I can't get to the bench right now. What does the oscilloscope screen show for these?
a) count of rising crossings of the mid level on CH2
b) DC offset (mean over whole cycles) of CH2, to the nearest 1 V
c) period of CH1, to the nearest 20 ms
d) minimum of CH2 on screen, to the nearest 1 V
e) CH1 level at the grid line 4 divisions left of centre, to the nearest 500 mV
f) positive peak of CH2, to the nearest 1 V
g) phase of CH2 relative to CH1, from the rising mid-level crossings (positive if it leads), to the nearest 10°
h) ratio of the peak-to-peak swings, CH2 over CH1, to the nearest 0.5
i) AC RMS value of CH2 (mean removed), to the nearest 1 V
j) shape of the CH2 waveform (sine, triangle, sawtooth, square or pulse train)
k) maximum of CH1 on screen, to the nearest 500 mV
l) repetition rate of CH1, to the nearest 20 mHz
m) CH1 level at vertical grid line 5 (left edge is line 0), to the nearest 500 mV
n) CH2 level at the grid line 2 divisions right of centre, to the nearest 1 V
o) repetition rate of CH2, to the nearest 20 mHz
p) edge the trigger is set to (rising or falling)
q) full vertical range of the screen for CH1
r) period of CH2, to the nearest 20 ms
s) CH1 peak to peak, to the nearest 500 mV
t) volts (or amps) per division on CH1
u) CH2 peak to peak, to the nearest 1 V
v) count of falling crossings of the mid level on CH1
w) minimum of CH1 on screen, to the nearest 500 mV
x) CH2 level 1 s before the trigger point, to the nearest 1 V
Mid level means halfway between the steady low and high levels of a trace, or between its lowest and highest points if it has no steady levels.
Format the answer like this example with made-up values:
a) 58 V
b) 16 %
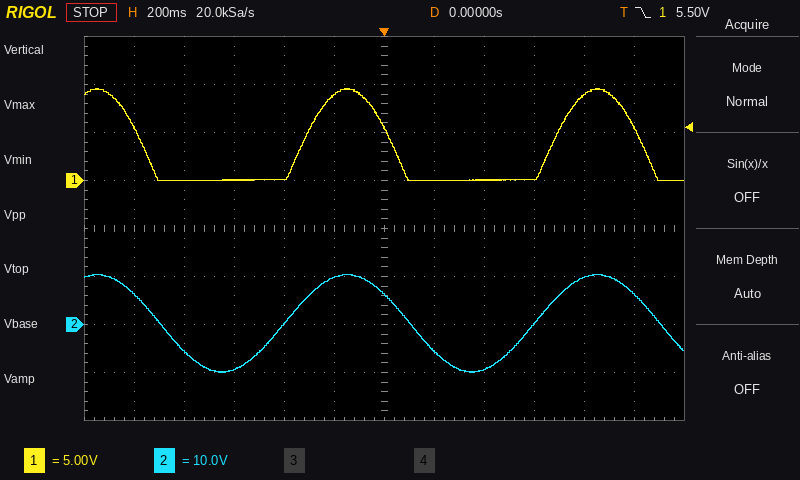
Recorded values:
a) 2
b) 0 V
c) 1.00 s
d) -10 V
e) 0.0 V
f) 10 V
g) +30°
h) 2.0
i) 7 V
j) sine
k) 9.5 V
l) 1.00 Hz
m) 9.0 V
n) -9 V
o) 1.00 Hz
p) falling
q) 40 V
r) 1.00 s
s) 9.5 V
t) 5 V
u) 20 V
v) 3
w) 0.0 V
x) 6 V
